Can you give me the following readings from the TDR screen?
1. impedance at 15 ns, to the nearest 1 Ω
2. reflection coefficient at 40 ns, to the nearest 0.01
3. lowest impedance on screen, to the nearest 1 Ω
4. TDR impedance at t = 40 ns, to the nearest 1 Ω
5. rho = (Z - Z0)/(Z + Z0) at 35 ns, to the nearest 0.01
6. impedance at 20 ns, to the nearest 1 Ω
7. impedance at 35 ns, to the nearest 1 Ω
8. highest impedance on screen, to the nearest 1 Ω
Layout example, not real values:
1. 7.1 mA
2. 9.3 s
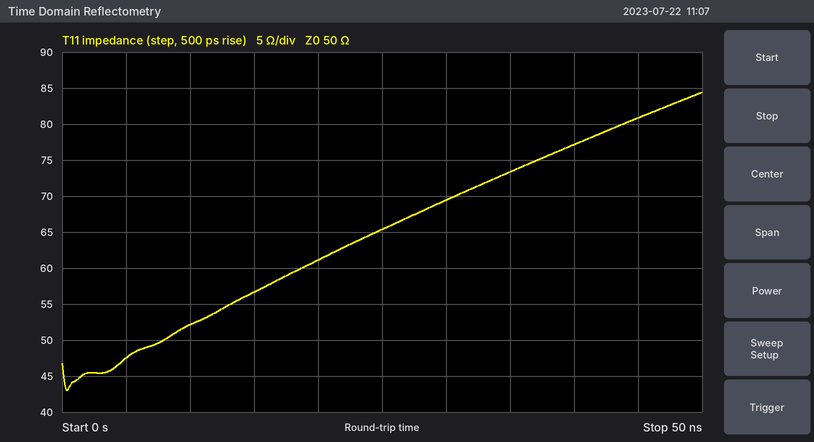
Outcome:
1. 57 Ω
2. +0.21
3. 43 Ω
4. 77 Ω
5. +0.19
6. 61 Ω
7. 73 Ω
8. 84 Ω
